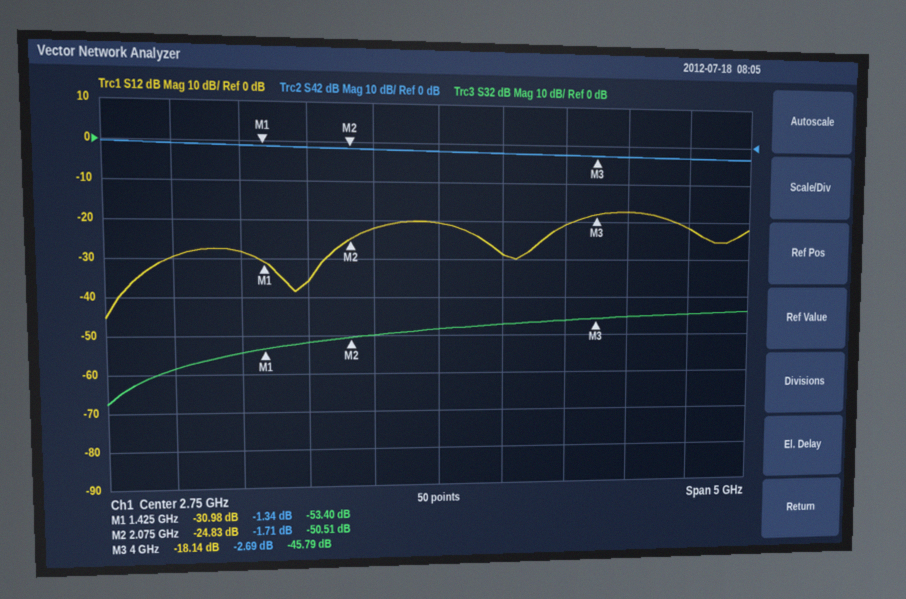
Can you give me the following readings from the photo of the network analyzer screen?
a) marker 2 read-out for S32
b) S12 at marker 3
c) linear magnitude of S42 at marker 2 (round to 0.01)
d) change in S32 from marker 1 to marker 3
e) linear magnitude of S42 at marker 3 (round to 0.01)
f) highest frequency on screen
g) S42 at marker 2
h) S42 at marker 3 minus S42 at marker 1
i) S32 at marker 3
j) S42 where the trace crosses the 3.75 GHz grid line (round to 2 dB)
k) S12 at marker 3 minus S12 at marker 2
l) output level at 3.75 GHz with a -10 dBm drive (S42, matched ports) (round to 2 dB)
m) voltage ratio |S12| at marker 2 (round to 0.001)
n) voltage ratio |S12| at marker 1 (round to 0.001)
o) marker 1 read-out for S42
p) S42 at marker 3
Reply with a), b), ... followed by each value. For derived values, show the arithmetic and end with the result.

a) -50.51 dB
b) -18.14 dB
c) 10^(-1.71/20) ≈ 0.82
d) -45.79 − (-53.4) = 7.61 dB
e) 10^(-2.69/20) ≈ 0.73
f) 5.25 GHz
g) -1.71 dB
h) -2.69 − (-1.34) = -1.35 dB
i) -45.79 dB
j) -2 dB
k) -18.14 − (-24.83) = 6.69 dB
l) -10 dBm + (-2 dB) = -12 dBm
m) 10^(-24.83/20) ≈ 0.057
n) 10^(-30.98/20) ≈ 0.028
o) -1.34 dB
p) -2.69 dB
